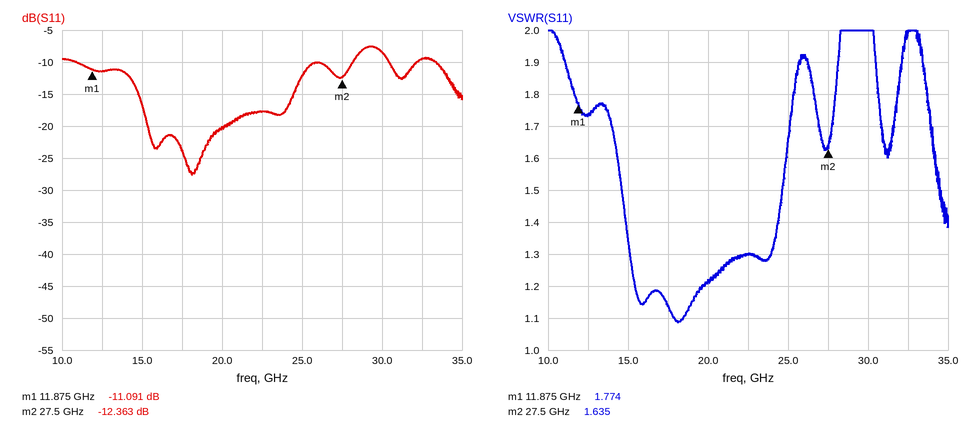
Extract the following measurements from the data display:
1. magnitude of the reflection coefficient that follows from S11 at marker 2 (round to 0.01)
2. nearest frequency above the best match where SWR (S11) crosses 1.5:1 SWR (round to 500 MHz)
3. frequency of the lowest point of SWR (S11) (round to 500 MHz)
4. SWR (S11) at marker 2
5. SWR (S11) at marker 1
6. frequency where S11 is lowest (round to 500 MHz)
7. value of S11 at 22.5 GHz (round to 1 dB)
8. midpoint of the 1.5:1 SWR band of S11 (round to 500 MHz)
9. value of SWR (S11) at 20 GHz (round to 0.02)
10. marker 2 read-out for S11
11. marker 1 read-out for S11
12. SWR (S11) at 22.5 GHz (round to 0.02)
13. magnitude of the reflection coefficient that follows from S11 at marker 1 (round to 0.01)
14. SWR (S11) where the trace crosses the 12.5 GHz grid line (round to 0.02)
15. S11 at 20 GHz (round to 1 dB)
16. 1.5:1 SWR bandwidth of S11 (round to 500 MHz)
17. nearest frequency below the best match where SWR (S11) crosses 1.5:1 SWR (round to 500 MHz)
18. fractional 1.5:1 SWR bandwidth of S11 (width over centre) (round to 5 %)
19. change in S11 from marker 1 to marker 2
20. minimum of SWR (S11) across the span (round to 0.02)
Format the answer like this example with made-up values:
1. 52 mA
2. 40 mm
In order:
1. 0.24
2. 24.5 GHz
3. 18.0 GHz
4. 1.635
5. 1.774
6. 18.0 GHz
7. -18 dB
8. 19.5 GHz
9. 1.22
10. -12.363 dB
11. -11.091 dB
12. 1.30
13. 0.28
14. 1.74
15. -20 dB
16. 10.0 GHz
17. 14.5 GHz
18. 50 %
19. -1.272 dB
20. 1.08
